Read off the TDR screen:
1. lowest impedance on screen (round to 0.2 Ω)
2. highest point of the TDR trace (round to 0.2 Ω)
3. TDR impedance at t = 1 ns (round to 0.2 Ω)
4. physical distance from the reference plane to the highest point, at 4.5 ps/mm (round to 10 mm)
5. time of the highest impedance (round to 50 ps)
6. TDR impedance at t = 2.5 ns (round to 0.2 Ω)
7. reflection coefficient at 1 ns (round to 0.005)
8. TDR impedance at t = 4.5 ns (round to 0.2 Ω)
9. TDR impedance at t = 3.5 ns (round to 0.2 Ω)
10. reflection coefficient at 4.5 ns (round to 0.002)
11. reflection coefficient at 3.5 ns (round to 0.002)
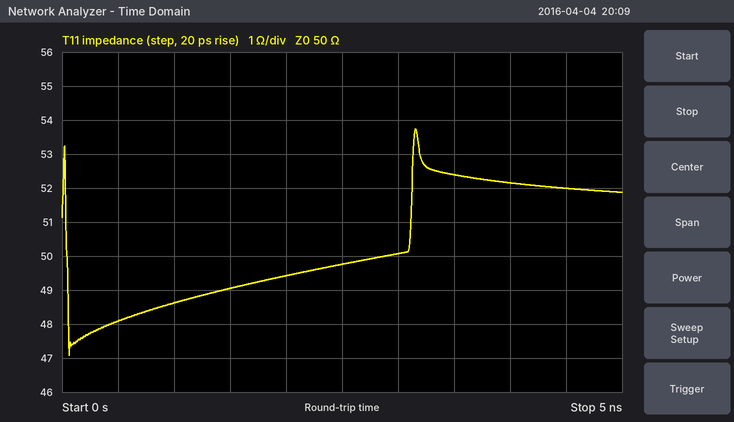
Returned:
47.0 Ω
53.8 Ω
48.6 Ω
350 mm
3.15 ns
49.8 Ω
-0.015
52.0 Ω
52.4 Ω
+0.020
+0.024
